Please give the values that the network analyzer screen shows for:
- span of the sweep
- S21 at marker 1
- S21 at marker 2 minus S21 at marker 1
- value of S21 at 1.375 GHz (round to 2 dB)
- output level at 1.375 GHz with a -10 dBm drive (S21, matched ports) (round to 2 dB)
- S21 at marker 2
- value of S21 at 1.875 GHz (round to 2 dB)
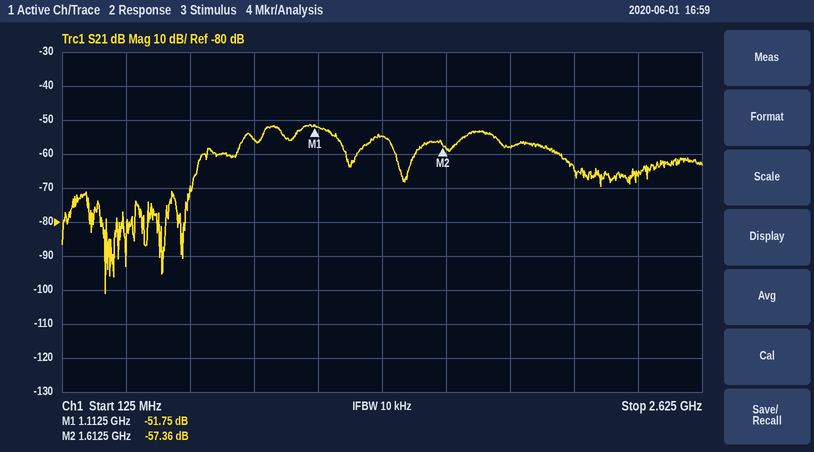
2.5 GHz
-51.75 dB
-5.61 dB
-54 dB
-64 dBm
-57.36 dB
-58 dB
